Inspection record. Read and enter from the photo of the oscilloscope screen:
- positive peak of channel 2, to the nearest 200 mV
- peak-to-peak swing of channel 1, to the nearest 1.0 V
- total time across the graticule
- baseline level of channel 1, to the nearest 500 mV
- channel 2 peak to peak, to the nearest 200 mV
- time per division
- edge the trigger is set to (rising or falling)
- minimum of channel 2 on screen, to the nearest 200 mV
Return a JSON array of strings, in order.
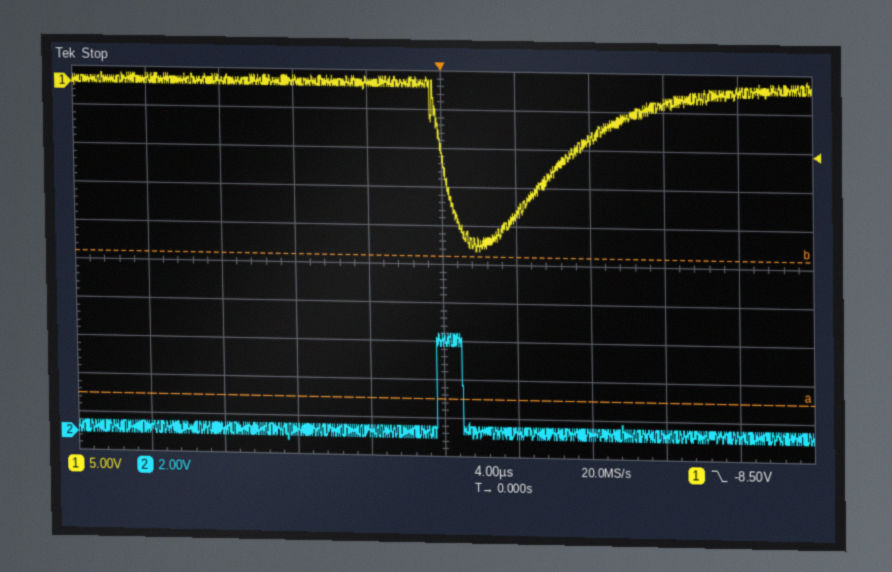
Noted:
["5.4 V", "22.0 V", "40 µs", "500 mV", "5.6 V", "4 µs", "falling", "-200 mV"]
